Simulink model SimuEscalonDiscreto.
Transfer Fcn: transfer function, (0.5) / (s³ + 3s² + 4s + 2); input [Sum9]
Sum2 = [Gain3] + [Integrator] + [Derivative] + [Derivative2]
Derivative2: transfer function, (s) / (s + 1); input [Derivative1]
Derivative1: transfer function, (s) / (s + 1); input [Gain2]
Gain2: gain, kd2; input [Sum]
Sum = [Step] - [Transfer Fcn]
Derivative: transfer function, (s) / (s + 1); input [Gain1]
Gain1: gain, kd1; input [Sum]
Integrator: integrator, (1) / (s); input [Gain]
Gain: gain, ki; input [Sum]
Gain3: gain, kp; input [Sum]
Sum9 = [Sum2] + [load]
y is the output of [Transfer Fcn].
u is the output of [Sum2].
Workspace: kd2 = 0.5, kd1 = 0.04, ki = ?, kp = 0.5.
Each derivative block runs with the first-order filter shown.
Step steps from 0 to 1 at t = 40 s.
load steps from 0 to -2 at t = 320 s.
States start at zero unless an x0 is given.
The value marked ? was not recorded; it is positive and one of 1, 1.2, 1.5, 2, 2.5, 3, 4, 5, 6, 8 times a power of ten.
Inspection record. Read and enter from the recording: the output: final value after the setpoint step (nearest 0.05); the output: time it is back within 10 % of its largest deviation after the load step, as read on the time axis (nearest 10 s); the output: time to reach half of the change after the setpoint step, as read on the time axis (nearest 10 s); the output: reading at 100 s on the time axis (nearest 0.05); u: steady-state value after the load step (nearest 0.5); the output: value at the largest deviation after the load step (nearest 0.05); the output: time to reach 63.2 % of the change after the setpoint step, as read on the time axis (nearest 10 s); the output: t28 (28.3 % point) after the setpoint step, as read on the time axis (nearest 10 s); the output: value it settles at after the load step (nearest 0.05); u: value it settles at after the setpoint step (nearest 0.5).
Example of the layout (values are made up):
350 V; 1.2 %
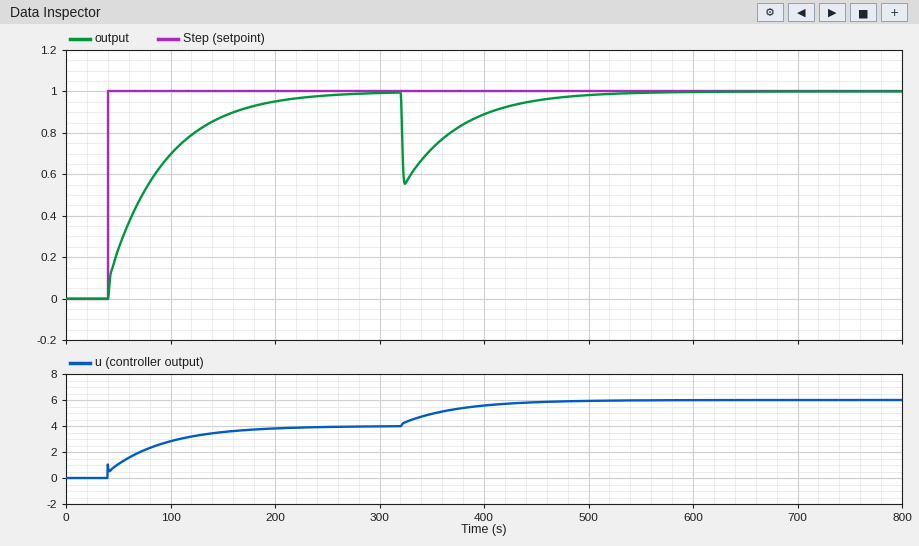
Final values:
1.00; 450 s; 70 s; 0.70; 6.0; 0.55; 90 s; 50 s; 1.00; 4.0
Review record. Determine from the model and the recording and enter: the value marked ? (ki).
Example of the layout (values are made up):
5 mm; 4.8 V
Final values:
0.08
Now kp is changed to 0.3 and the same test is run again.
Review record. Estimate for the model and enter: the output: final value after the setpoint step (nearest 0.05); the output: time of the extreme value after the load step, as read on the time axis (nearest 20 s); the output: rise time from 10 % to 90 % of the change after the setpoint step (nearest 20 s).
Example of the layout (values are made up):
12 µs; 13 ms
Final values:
1.00; 320 s; 120 s
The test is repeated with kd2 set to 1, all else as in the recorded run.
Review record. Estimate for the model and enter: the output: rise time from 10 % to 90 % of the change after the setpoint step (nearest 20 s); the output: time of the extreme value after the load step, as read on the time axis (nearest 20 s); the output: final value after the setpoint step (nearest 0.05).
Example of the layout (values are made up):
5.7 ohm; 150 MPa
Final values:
120 s; 320 s; 1.00
